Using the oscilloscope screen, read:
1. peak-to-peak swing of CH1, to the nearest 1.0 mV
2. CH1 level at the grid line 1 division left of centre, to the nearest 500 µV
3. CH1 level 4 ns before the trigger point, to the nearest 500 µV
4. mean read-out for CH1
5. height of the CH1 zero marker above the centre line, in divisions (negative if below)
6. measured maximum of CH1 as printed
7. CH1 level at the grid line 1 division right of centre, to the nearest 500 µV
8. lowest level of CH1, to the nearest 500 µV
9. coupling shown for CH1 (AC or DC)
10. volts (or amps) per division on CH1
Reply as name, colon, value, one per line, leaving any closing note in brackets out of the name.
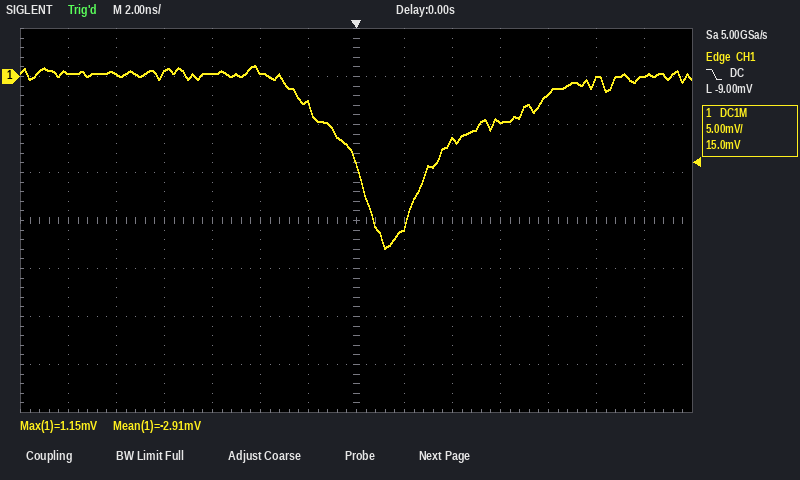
peak-to-peak swing of CH1, to the nearest 1.0 mV: 19.0 mV
CH1 level at the grid line 1 division left of centre, to the nearest 500 µV: -3.0 mV
CH1 level 4 ns before the trigger point, to the nearest 500 µV: 500 µV
mean read-out for CH1: -2.91 mV
height of the CH1 zero marker above the centre line, in divisions: +3.0 div
measured maximum of CH1 as printed: 1.15 mV
CH1 level at the grid line 1 division right of centre, to the nearest 500 µV: -15.5 mV
lowest level of CH1, to the nearest 500 µV: -18.0 mV
coupling shown for CH1: DC
volts (or amps) per division on CH1: 5 mV
